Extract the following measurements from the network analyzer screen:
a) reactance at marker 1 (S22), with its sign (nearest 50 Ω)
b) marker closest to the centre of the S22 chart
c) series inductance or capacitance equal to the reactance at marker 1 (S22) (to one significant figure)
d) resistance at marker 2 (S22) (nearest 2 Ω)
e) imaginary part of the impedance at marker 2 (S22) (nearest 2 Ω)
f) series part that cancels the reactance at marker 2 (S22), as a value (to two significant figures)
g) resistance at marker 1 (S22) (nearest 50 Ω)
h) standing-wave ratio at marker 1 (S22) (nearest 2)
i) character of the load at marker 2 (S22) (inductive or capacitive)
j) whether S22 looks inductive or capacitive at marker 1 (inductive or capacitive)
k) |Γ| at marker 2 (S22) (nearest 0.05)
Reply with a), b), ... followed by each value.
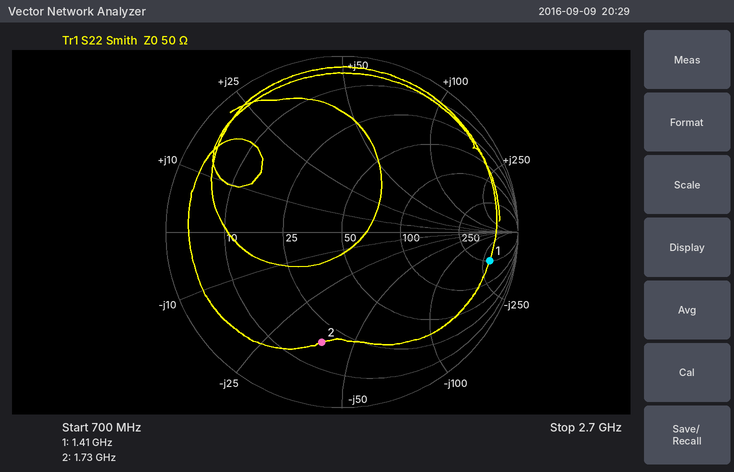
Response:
a) -300 Ω
b) marker 2
c) 400 fF
d) 18 Ω
e) -38 Ω
f) 3.5 nH
g) 250 Ω
h) 12
i) capacitive
j) capacitive
k) 0.65
